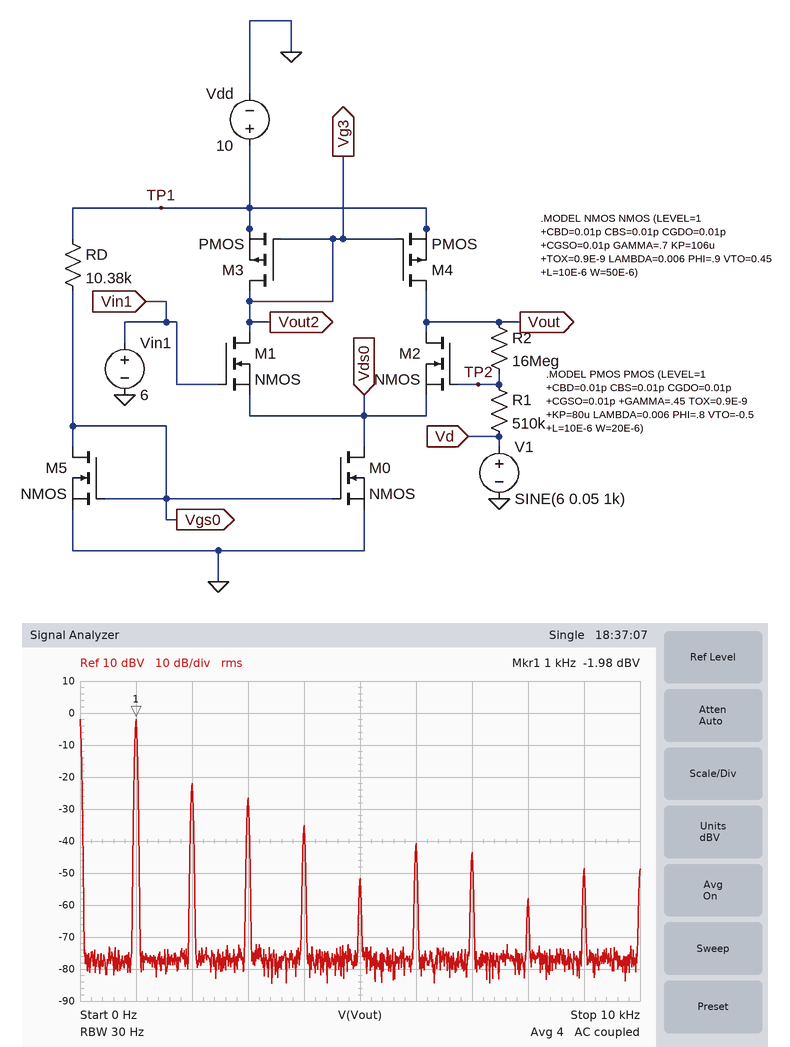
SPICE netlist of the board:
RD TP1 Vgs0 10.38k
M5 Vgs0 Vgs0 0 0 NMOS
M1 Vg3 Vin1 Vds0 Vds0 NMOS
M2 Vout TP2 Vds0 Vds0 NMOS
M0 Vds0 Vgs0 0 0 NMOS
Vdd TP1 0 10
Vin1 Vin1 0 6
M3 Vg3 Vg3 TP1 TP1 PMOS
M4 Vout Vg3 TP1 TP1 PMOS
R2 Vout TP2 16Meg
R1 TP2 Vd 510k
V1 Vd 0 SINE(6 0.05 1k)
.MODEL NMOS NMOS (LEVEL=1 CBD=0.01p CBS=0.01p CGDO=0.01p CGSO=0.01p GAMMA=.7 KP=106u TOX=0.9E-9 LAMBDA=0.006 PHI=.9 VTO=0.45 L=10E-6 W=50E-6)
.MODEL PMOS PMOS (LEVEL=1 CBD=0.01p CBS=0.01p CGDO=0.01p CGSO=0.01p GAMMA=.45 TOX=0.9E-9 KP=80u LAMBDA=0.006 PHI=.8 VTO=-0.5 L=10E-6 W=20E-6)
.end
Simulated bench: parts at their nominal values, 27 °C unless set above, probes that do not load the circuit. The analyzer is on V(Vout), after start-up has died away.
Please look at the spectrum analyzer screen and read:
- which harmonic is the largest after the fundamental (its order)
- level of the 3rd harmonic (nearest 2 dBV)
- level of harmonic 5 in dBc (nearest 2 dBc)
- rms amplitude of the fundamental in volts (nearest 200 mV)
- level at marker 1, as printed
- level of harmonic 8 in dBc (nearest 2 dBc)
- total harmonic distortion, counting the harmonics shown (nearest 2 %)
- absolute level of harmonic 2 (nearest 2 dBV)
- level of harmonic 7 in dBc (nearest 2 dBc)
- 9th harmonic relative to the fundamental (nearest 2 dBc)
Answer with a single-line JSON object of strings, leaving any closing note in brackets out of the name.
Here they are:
{"which harmonic is the largest after the fundamental": "2", "level of the 3rd harmonic": "-26 dBV", "level of harmonic 5 in dBc": "-50 dBc", "rms amplitude of the fundamental in volts": "800 mV", "level at marker 1, as printed": "-1.98 dBV", "level of harmonic 8 in dBc": "-56 dBc", "total harmonic distortion, counting the harmonics shown": "12 %", "absolute level of harmonic 2": "-22 dBV", "level of harmonic 7 in dBc": "-42 dBc", "9th harmonic relative to the fundamental": "-46 dBc"}
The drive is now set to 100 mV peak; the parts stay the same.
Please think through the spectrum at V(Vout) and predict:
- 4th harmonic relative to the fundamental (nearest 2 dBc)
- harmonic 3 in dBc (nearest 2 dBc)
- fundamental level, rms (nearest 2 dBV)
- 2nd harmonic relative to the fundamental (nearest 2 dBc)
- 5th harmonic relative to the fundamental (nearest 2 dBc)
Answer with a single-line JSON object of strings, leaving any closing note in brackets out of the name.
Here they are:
{"4th harmonic relative to the fundamental": "-26 dBc", "harmonic 3 in dBc": "-18 dBc", "fundamental level, rms": "2 dBV", "2nd harmonic relative to the fundamental": "-16 dBc", "5th harmonic relative to the fundamental": "-32 dBc"}
